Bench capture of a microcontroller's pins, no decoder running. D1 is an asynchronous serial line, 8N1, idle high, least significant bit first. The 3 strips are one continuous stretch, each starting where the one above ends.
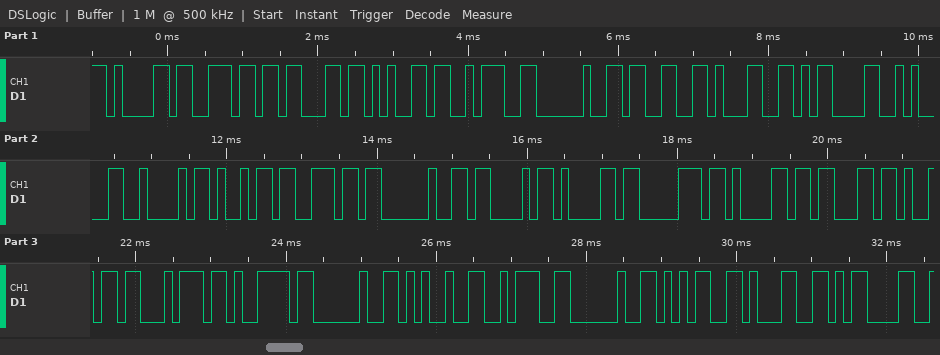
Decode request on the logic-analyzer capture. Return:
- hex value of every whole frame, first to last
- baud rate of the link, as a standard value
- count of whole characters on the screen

0x61 0x6E 0x63 0x65 0x3A 0x20 0x33 0x31 0x0D 0x0A 0x42 0x69 0x6E 0x20 0x43 0x61 0x70 0x61 0x63 0x69 0x74 0x79 0x20 0x25 0x3A 0x20 0x35 0x31 0x0D
9600 baud
29
